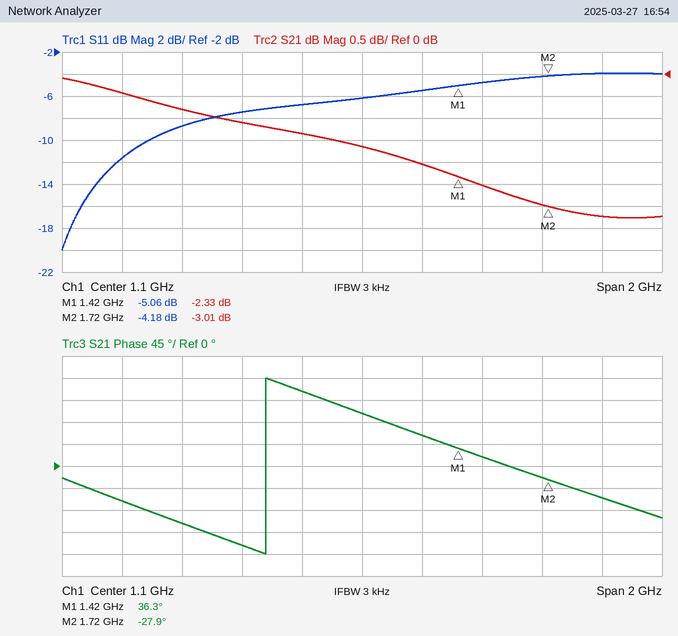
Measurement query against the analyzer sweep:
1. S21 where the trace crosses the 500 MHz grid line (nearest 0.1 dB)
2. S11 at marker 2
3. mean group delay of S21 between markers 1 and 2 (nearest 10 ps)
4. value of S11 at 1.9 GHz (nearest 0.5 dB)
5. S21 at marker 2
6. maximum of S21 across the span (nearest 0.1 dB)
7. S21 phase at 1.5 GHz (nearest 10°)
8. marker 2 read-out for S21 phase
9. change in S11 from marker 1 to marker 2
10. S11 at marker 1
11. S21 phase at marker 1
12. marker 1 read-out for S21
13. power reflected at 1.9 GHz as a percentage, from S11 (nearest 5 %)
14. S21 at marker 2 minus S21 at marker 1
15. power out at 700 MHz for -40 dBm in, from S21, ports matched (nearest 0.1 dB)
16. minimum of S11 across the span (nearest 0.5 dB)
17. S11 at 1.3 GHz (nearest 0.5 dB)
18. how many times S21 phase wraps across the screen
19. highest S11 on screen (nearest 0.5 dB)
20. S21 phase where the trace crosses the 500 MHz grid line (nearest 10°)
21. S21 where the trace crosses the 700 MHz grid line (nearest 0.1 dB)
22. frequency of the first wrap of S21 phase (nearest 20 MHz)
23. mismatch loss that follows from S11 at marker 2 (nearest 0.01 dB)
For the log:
-0.8 dB
-4.18 dB
590 ps
-4.0 dB
-3.01 dB
-0.1 dB
20°
-27.9°
0.88 dB
-5.06 dB
36.3°
-2.33 dB
40 %
-0.68 dB
-41.1 dBm
-20.0 dB
-5.5 dB
1
-4.0 dB
-120°
-1.1 dB
780 MHz
2.09 dB
